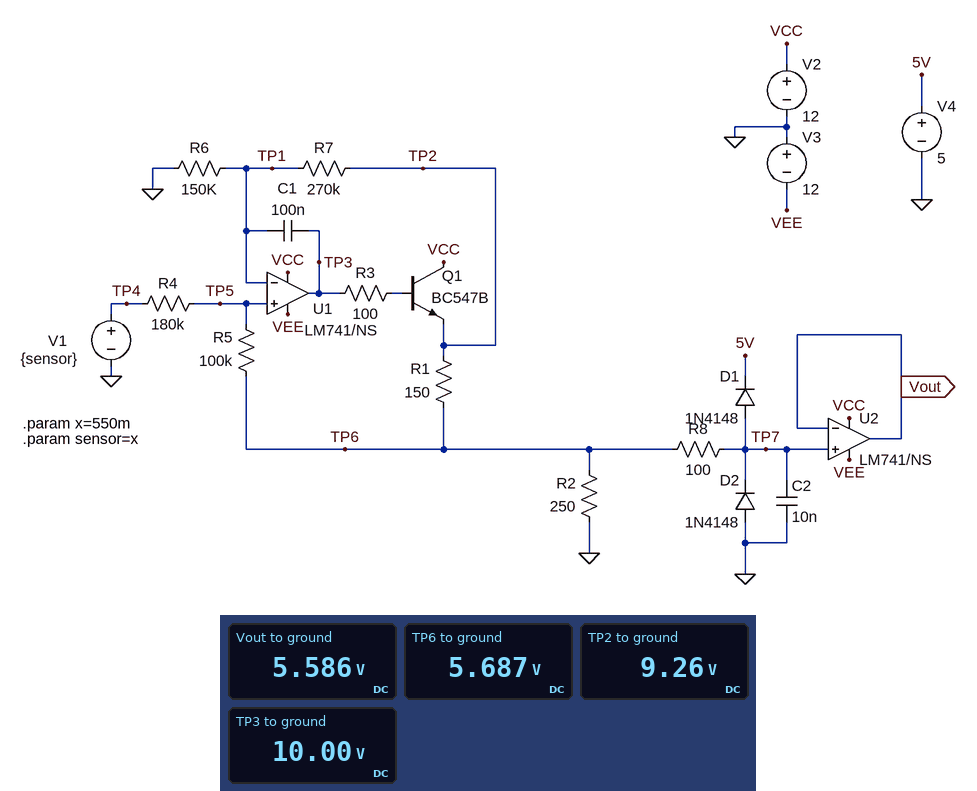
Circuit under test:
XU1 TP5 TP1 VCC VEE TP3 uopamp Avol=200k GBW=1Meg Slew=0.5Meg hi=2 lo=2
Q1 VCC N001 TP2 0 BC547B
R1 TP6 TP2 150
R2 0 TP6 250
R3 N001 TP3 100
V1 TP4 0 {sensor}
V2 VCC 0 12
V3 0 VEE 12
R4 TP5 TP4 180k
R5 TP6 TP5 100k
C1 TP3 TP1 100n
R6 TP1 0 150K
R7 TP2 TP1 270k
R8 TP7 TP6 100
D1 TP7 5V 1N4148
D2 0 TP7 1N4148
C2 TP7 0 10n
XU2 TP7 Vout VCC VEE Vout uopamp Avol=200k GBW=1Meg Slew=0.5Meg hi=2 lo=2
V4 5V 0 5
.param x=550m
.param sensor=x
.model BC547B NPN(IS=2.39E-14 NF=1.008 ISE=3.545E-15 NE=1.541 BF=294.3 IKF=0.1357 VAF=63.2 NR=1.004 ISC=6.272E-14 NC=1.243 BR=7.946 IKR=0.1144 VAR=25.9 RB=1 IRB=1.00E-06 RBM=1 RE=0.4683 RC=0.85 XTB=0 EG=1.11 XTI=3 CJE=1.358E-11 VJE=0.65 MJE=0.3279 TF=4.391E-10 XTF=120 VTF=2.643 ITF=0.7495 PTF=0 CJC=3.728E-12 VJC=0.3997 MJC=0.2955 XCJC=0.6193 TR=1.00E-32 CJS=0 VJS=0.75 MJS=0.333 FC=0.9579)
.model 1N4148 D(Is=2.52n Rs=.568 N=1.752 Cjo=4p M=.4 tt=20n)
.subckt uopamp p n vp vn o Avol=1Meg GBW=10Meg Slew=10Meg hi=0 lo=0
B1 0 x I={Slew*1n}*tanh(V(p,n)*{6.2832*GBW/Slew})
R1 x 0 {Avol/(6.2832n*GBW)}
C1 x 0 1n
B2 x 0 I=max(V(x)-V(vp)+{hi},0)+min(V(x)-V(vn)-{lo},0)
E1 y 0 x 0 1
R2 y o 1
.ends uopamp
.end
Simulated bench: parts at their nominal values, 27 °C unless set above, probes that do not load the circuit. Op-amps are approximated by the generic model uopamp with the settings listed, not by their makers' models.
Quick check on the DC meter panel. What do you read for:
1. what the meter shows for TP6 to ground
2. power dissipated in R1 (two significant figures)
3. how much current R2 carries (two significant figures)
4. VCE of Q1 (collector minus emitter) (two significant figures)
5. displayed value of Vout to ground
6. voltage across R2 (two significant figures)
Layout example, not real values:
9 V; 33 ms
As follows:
5.687 V; 85 mW; 23 mA; 2.7 V; 5.586 V; 5.7 V
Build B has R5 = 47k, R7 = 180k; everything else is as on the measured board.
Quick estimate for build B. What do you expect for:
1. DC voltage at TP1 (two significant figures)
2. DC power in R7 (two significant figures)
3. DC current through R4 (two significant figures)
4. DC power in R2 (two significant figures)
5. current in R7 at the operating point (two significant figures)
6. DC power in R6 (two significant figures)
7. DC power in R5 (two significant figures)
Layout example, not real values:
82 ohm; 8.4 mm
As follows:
4.2 V; 140 µW; 23 µA; 130 mW; 28 µA; 120 µW; 24 µW
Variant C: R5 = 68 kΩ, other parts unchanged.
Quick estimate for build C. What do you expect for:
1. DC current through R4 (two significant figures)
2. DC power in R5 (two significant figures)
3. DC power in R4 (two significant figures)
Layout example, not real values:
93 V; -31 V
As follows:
21 µA; 29 µW; 77 µW
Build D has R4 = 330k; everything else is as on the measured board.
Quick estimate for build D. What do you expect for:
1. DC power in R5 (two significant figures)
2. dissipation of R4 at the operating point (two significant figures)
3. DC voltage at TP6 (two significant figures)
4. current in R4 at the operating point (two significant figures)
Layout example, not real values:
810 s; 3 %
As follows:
14 µW; 47 µW; 5.7 V; 12 µA
